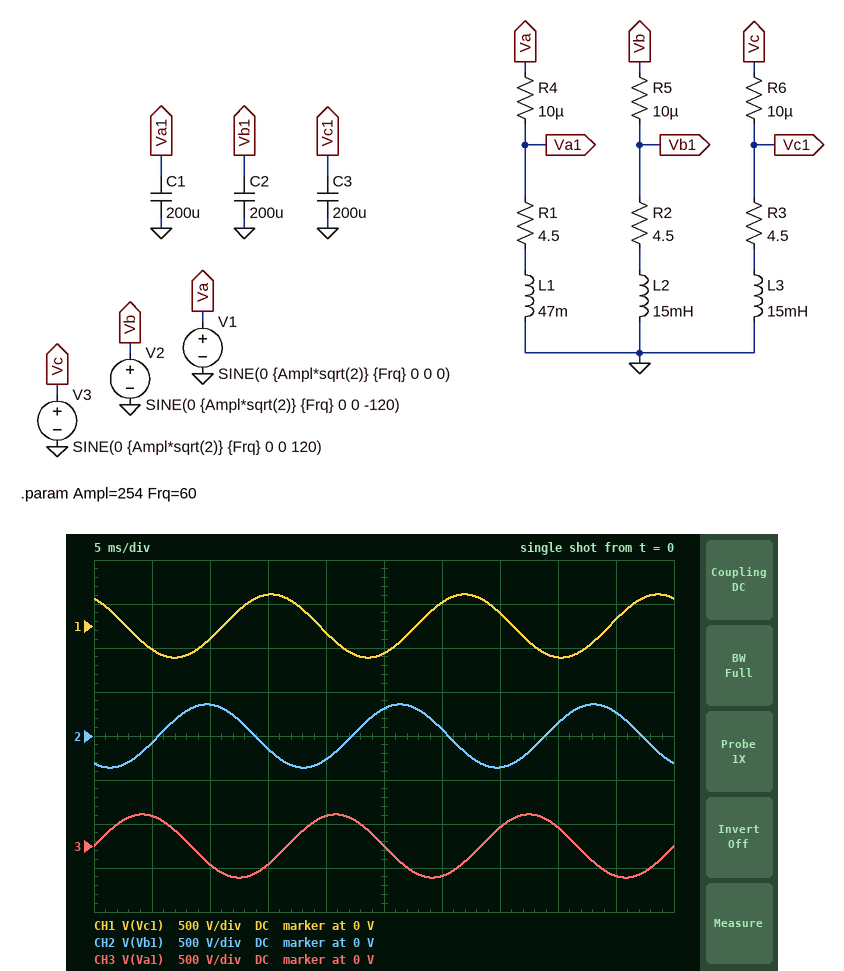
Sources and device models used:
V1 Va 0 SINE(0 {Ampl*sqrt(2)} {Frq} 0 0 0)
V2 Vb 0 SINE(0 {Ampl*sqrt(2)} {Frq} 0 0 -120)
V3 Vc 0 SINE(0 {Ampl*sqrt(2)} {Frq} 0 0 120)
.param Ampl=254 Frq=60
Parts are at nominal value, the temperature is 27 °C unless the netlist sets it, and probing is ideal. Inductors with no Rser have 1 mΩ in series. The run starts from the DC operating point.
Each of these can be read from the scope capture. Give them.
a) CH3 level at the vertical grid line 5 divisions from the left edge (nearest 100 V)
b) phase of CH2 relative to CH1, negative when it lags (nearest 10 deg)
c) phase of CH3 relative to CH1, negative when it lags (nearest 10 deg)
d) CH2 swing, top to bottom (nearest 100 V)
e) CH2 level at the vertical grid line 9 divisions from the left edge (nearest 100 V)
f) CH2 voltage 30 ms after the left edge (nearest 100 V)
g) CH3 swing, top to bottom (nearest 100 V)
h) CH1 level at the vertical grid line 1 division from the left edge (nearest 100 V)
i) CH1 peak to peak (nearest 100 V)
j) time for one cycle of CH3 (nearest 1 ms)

0 V
120 deg
-120 deg
700 V
300 V
100 V
700 V
-300 V
700 V
17 ms
